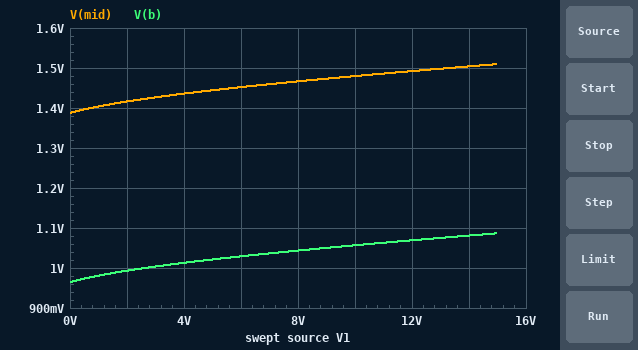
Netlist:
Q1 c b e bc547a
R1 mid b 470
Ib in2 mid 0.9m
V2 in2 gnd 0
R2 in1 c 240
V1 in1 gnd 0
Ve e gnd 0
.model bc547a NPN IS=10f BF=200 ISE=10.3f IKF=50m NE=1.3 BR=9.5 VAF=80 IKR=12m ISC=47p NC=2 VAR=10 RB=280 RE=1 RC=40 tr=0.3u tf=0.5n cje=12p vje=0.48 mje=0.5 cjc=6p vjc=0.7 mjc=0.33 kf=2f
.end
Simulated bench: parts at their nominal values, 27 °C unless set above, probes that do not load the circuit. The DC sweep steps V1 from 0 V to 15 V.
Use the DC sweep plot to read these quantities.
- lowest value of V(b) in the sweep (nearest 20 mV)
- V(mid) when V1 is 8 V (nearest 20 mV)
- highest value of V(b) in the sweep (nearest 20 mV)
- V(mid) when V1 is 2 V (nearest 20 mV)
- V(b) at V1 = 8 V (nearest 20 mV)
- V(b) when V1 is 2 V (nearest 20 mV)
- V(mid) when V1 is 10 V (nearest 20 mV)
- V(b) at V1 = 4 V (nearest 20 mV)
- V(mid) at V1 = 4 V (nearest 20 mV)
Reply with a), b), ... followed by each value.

a) 960 mV
b) 1.46 V
c) 1.08 V
d) 1.42 V
e) 1.04 V
f) 1.00 V
g) 1.48 V
h) 1.02 V
i) 1.44 V
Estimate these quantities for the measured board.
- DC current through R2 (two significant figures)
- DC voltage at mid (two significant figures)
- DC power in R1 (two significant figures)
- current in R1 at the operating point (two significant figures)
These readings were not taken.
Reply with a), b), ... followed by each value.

a) 18 µA
b) 1.4 V
c) 380 µW
d) 900 µA
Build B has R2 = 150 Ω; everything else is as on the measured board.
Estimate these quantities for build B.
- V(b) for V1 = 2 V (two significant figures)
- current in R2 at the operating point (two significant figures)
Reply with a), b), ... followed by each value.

a) 1.0 V
b) 27 µA
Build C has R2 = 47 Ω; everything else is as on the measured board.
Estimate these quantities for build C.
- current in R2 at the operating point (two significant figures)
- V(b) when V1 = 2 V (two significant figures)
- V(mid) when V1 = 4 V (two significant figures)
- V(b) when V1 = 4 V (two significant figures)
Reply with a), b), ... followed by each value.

a) 57 µA
b) 1.0 V
c) 1.5 V
d) 1.1 V
